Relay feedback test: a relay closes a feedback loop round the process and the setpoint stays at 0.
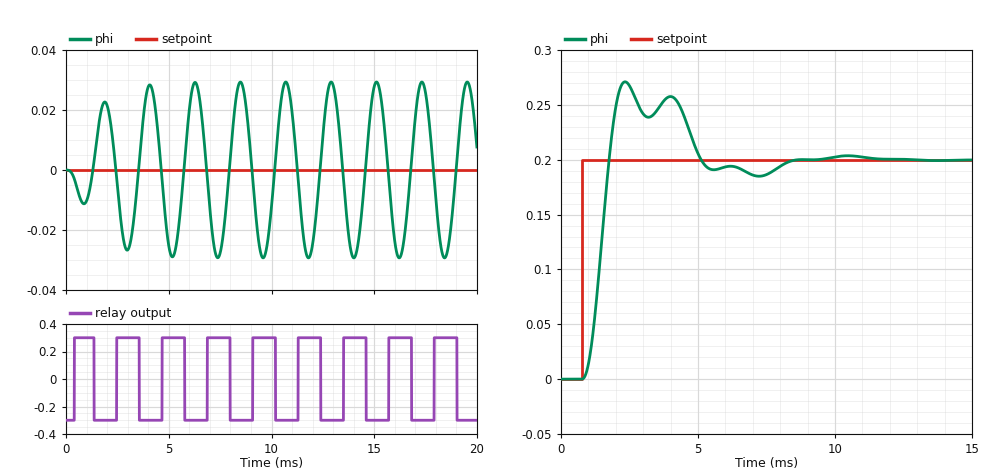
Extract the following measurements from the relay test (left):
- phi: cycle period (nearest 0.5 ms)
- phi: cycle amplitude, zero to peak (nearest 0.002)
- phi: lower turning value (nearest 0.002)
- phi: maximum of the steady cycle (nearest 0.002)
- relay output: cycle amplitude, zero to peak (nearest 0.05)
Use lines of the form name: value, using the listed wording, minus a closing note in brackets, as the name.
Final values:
phi: cycle period: 2.0 ms
phi: cycle amplitude, zero to peak: 0.030
phi: lower turning value: -0.030
phi: maximum of the steady cycle: 0.030
relay output: cycle amplitude, zero to peak: 0.30
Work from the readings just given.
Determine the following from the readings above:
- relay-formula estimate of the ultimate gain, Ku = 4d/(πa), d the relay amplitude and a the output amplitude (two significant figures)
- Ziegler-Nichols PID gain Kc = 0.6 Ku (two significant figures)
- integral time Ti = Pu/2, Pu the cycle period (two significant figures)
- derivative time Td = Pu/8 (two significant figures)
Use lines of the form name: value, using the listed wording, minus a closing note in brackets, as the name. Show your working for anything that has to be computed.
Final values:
relay-formula estimate of the ultimate gain, Ku = 4d/(πa), d the relay amplitude and a the output amplitude: 4 × 0.3 / (π × 0.03) = 13
Ziegler-Nichols PID gain Kc = 0.6 Ku: 0.6 × 13 = 7.8
integral time Ti = Pu/2, Pu the cycle period: 2 / 2 = 1.0 ms
derivative time Td = Pu/8: 2 / 8 = 0.25 ms
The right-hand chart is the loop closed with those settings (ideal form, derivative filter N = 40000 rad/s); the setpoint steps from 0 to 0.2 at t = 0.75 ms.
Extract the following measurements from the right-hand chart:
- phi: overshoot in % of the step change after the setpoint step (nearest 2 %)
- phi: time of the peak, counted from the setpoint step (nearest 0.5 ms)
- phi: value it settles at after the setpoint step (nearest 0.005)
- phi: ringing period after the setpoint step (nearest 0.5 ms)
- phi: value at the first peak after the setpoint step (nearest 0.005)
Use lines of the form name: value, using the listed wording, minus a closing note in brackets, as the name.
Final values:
phi: overshoot in % of the step change after the setpoint step: 36 %
phi: time of the peak, counted from the setpoint step: 1.5 ms
phi: value it settles at after the setpoint step: 0.200
phi: ringing period after the setpoint step: 1.5 ms
phi: value at the first peak after the setpoint step: 0.270
